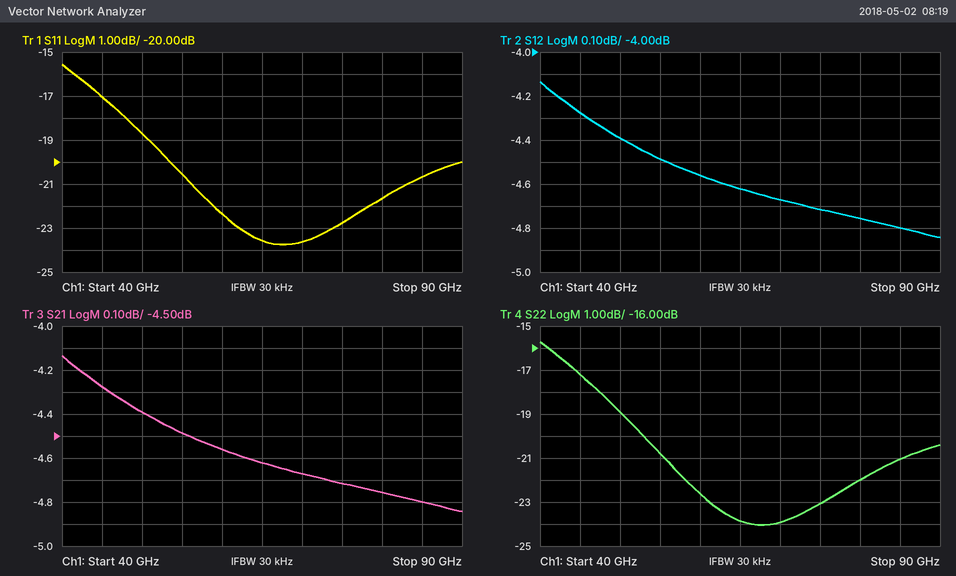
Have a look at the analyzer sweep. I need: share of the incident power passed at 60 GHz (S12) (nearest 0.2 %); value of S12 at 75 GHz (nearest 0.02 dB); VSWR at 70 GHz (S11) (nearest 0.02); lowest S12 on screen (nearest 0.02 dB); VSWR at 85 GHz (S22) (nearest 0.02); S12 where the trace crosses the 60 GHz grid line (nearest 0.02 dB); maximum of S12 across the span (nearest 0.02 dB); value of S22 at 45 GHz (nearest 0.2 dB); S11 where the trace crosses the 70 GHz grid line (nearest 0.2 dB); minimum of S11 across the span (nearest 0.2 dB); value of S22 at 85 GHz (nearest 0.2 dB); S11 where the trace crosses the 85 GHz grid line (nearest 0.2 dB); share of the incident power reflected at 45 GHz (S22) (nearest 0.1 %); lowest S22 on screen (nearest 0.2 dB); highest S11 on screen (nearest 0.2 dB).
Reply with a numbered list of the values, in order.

1. 35.0 %
2. -4.72 dB
3. 1.14
4. -4.84 dB
5. 1.20
6. -4.56 dB
7. -4.14 dB
8. -17.2 dB
9. -23.6 dB
10. -23.8 dB
11. -21.0 dB
12. -20.6 dB
13. 1.9 %
14. -24.0 dB
15. -15.6 dB
